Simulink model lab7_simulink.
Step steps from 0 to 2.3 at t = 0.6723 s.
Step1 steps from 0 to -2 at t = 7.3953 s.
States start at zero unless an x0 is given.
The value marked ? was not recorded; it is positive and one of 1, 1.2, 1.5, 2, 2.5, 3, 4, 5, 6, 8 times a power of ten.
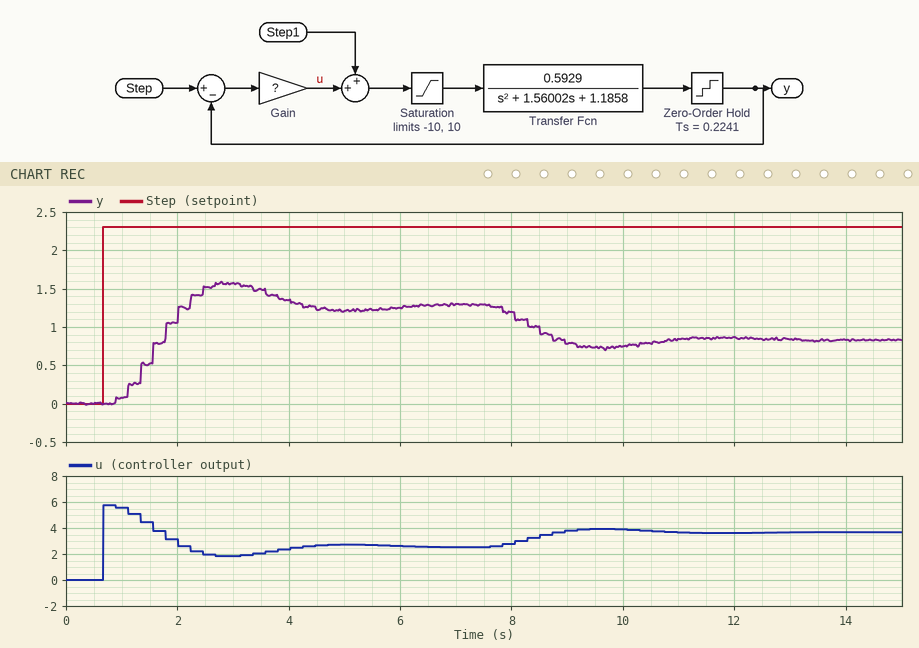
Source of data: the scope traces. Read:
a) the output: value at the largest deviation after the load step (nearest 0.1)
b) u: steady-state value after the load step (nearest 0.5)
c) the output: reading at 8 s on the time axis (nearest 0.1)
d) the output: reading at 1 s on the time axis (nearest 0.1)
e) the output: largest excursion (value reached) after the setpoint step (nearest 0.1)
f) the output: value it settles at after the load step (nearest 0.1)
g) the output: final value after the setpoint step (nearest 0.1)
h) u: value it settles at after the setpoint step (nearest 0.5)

0.7
3.5
1.2
0.1
1.6
0.8
1.3
2.5
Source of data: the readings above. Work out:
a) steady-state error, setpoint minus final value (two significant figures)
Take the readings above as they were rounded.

1.00
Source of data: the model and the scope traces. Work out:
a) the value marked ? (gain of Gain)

2.5
